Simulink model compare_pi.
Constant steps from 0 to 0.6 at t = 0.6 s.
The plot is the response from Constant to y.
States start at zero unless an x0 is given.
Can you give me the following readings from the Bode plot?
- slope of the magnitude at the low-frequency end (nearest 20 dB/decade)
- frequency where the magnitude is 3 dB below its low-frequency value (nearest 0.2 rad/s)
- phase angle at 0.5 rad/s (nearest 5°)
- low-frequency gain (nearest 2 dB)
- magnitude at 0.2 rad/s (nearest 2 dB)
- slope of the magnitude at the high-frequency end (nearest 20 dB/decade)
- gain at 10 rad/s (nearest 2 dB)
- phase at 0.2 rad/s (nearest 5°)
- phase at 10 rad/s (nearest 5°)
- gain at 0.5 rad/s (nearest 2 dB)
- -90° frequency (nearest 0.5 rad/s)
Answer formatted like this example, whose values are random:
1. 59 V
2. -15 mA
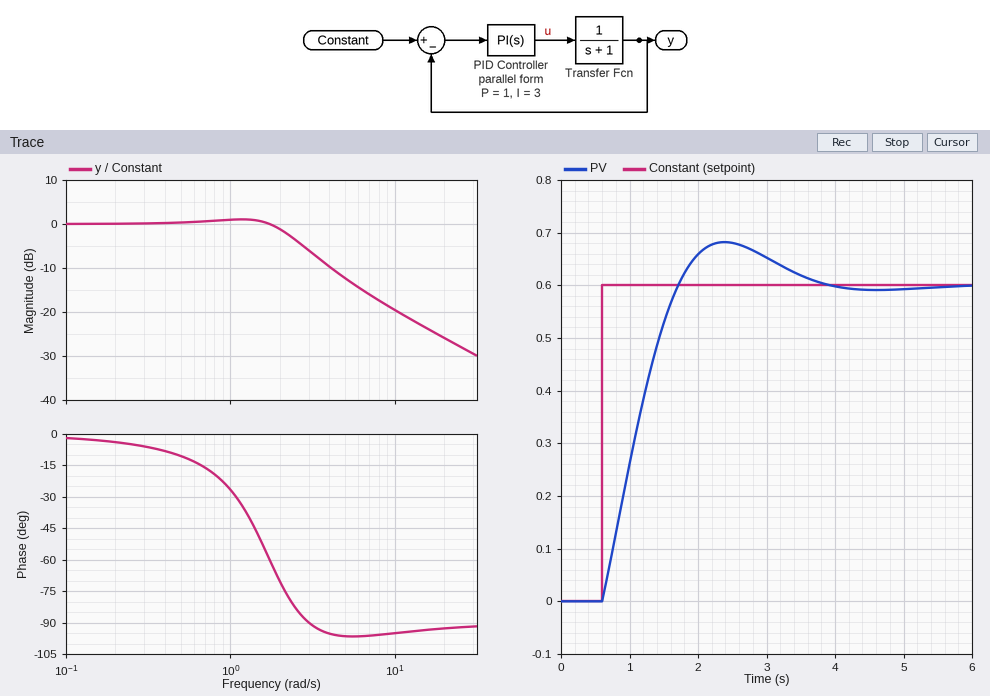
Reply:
1. 0 dB/decade
2. 2.4 rad/s
3. -10°
4. 0 dB
5. 0 dB
6. -20 dB/decade
7. -20 dB
8. -5°
9. -95°
10. 0 dB
11. 3.0 rad/s
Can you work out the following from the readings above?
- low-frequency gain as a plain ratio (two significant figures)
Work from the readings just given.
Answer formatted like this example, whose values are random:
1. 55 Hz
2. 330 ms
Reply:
1. 1.0
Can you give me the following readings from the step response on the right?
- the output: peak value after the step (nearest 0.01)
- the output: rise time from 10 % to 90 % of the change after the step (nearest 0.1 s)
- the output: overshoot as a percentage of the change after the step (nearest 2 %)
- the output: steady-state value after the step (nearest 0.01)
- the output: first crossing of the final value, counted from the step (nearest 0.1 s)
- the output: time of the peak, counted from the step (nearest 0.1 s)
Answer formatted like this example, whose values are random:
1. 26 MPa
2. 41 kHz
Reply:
1. 0.68
2. 0.8 s
3. 14 %
4. 0.60
5. 1.1 s
6. 1.8 s
